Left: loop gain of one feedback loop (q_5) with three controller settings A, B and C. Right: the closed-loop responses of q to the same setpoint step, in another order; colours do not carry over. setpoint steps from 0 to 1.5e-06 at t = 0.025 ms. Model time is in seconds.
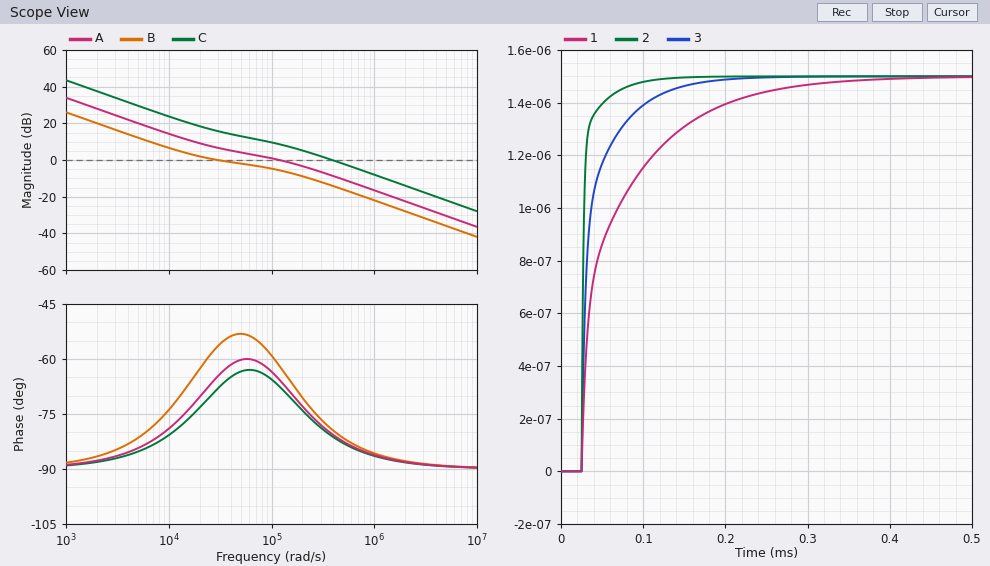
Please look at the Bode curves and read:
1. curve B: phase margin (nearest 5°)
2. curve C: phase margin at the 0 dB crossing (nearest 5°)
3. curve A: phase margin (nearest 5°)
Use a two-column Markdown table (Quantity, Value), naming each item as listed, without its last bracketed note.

| Quantity | Value |
|---|---|
| curve B: phase margin | 125° |
| curve C: phase margin at the 0 dB crossing | 100° |
| curve A: phase margin | 115° |
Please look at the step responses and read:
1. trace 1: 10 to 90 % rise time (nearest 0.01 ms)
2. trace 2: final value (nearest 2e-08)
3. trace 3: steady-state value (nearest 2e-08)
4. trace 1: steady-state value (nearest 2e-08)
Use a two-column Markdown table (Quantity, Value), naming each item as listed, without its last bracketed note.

| Quantity | Value |
|---|---|
| trace 1: 10 to 90 % rise time | 0.14 ms |
| trace 2: final value | 0.00000150 |
| trace 3: steady-state value | 0.00000150 |
| trace 1: steady-state value | 0.00000150 |
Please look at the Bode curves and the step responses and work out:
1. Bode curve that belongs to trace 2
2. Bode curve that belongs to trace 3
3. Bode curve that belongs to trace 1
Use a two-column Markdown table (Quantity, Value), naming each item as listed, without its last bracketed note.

| Quantity | Value |
|---|---|
| Bode curve that belongs to trace 2 | C |
| Bode curve that belongs to trace 3 | A |
| Bode curve that belongs to trace 1 | B |
